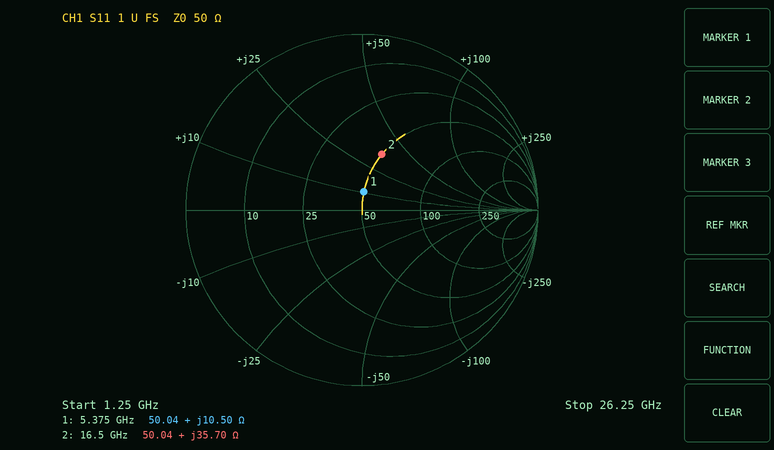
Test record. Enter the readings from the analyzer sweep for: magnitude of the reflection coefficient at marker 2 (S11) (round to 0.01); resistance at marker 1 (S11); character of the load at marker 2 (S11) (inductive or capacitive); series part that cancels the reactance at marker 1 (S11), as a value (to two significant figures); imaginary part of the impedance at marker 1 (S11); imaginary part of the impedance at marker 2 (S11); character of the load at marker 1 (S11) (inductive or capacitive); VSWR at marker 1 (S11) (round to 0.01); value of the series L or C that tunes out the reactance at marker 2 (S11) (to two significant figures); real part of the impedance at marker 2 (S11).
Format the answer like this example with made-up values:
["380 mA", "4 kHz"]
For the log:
["0.34", "50.04 Ω", "inductive", "2.8 pF", "+10.50 Ω", "+35.70 Ω", "inductive", "1.23", "270 fF", "50.04 Ω"]
